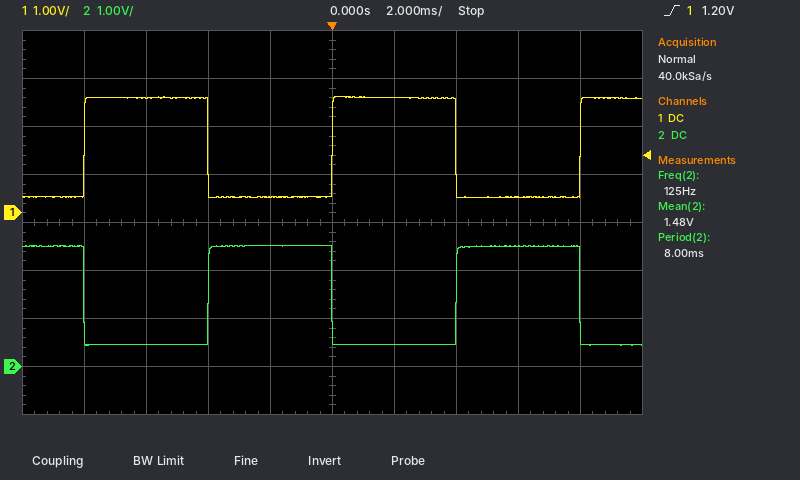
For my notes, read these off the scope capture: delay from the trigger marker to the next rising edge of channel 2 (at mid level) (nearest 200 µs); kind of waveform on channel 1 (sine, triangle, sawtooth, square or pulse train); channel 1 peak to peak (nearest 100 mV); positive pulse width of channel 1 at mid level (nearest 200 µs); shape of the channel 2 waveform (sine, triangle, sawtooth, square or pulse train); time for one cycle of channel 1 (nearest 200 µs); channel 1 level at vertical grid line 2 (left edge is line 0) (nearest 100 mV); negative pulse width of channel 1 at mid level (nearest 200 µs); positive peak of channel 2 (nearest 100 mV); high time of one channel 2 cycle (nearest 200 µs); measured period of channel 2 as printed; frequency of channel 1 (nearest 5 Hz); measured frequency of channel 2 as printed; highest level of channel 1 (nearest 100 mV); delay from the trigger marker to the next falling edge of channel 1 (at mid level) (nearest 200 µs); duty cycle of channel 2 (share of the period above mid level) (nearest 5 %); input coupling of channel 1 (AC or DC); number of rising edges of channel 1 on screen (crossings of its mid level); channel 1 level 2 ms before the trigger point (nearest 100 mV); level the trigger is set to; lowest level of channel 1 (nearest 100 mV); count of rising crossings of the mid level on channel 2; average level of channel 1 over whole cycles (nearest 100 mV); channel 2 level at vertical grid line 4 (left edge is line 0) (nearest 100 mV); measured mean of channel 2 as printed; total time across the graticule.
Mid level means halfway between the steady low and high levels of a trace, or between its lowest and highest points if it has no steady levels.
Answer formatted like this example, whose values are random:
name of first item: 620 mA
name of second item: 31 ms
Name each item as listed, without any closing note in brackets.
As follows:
delay from the trigger marker to the next rising edge of channel 2 (at mid level): 4.0 ms
kind of waveform on channel 1: square
channel 1 peak to peak: 2.1 V
positive pulse width of channel 1 at mid level: 4.0 ms
shape of the channel 2 waveform: square
time for one cycle of channel 1: 8.0 ms
channel 1 level at vertical grid line 2 (left edge is line 0): 2.4 V
negative pulse width of channel 1 at mid level: 4.0 ms
positive peak of channel 2: 2.5 V
high time of one channel 2 cycle: 4.0 ms
measured period of channel 2 as printed: 8.00 ms
frequency of channel 1: 125 Hz
measured frequency of channel 2 as printed: 125 Hz
highest level of channel 1: 2.4 V
delay from the trigger marker to the next falling edge of channel 1 (at mid level): 4.0 ms
duty cycle of channel 2 (share of the period above mid level): 50 %
input coupling of channel 1: DC
number of rising edges of channel 1 on screen: 3
channel 1 level 2 ms before the trigger point: 300 mV
level the trigger is set to: 1.20 V
lowest level of channel 1: 300 mV
count of rising crossings of the mid level on channel 2: 2
average level of channel 1 over whole cycles: 1.4 V
channel 2 level at vertical grid line 4 (left edge is line 0): 2.5 V
measured mean of channel 2 as printed: 1.48 V
total time across the graticule: 20 ms
